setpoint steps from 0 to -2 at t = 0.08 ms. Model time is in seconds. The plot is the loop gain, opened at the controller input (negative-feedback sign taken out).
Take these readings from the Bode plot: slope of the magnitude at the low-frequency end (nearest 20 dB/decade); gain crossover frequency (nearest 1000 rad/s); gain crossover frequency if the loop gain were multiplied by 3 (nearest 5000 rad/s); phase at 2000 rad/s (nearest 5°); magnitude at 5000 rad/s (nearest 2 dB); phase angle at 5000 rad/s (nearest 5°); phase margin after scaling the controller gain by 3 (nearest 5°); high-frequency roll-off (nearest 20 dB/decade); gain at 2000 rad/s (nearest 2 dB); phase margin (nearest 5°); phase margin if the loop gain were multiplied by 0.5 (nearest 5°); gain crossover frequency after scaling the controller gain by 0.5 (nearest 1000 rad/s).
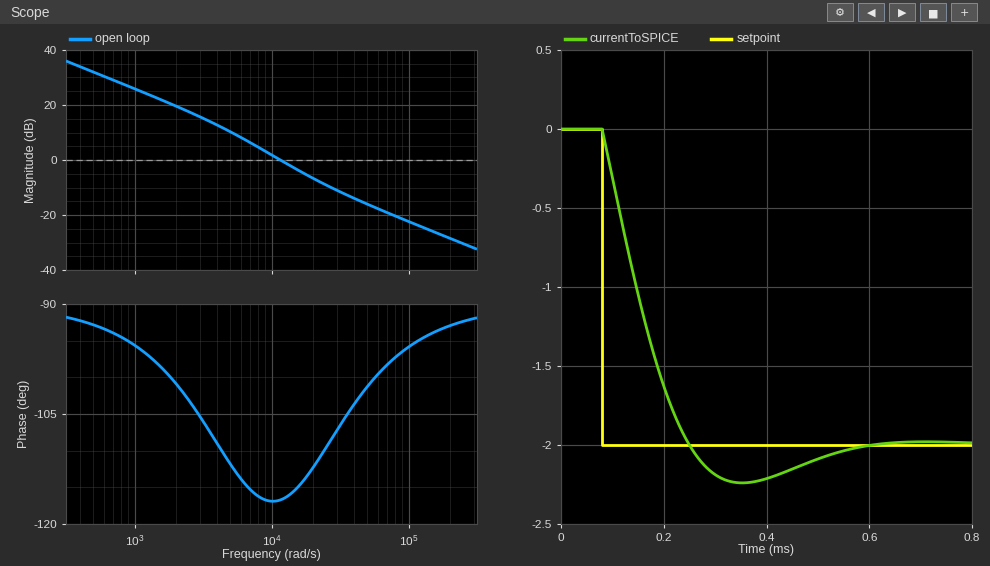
-20 dB/decade
12000 rad/s
25000 rad/s
-100°
10 dB
-110°
70°
-20 dB/decade
20 dB
65°
65°
7000 rad/s
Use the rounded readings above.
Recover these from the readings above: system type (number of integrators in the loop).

1
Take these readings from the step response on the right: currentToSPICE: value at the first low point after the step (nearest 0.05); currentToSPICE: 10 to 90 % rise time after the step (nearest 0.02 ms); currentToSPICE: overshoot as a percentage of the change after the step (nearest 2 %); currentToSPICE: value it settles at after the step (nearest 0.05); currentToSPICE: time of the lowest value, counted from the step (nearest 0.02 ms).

-2.25
0.12 ms
12 %
-2.00
0.28 ms
